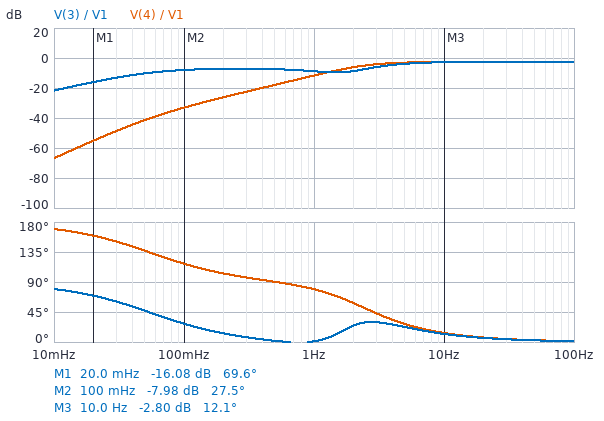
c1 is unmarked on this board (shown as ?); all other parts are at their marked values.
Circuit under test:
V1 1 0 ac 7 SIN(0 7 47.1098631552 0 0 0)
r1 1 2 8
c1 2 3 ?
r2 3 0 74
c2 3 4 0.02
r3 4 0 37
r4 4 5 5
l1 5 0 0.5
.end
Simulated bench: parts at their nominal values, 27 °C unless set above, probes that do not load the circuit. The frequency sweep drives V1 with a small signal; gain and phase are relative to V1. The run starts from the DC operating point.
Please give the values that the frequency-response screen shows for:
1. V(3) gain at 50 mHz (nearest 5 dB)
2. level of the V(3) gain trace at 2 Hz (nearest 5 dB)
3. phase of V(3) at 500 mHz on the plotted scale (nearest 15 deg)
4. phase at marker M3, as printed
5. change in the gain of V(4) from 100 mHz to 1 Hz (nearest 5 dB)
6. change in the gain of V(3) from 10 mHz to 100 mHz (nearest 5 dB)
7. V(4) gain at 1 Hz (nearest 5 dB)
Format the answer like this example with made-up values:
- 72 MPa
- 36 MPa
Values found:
- -10 dB
- -10 dB
- 0 deg
- 12.1 deg
- 20 dB
- 15 dB
- -10 dB
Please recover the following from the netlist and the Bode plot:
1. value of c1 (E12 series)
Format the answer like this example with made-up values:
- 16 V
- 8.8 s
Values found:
- 18 mF
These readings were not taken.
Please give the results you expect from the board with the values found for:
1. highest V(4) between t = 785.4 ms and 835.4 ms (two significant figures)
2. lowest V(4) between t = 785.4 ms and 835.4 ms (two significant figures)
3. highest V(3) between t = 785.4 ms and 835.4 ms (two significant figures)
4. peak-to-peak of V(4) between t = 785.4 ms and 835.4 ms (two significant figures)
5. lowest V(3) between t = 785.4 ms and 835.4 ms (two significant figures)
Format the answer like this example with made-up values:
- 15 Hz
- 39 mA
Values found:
- 5.3 V
- -5.3 V
- 5.3 V
- 11 V
- -5.3 V
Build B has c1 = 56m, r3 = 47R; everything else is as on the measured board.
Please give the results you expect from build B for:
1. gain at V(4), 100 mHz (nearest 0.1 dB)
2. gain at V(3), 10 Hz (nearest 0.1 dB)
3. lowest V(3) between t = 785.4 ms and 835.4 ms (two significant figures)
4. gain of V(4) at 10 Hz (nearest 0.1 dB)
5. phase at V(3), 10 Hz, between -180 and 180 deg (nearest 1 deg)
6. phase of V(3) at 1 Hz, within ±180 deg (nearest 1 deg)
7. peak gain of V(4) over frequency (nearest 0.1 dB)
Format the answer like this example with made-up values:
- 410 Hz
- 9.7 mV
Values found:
- -28.4 dB
- -2.6 dB
- -5.5 V
- -2.4 dB
- 11 deg
- -14 deg
- -2.1 dB
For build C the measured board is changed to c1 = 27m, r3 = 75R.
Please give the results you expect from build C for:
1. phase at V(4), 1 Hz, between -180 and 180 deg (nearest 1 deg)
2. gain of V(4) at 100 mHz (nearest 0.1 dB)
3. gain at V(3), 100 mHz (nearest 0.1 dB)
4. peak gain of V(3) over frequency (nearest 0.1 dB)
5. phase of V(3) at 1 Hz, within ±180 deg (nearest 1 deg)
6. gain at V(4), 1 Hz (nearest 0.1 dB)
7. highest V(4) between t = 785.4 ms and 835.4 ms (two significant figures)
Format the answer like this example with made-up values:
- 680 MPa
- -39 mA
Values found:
- 73 deg
- -30.6 dB
- -6.0 dB
- -1.7 dB
- -4 deg
- -10.1 dB
- 5.8 V
